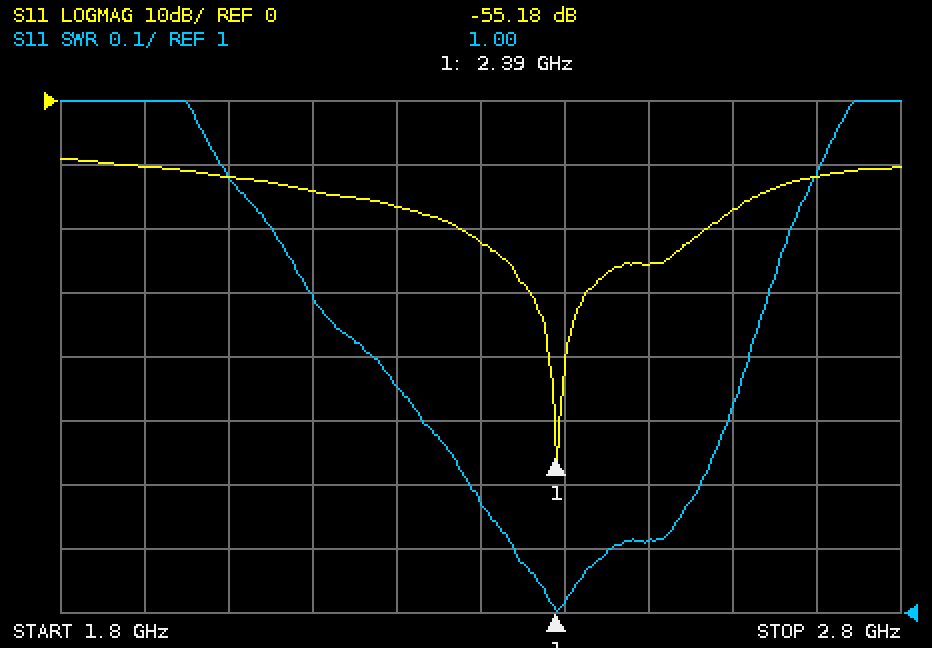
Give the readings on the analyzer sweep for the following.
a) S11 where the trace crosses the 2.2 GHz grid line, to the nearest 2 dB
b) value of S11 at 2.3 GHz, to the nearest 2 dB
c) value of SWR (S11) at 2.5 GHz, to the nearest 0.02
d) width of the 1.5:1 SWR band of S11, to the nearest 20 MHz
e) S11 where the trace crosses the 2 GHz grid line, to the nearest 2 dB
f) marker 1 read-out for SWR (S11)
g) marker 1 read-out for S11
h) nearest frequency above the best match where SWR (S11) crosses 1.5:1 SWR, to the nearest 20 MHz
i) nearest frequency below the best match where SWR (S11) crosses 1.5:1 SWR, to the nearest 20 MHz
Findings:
-16 dB
-22 dB
1.12
540 MHz
-12 dB
1.00
-55.18 dB
2.64 GHz
2.10 GHz
